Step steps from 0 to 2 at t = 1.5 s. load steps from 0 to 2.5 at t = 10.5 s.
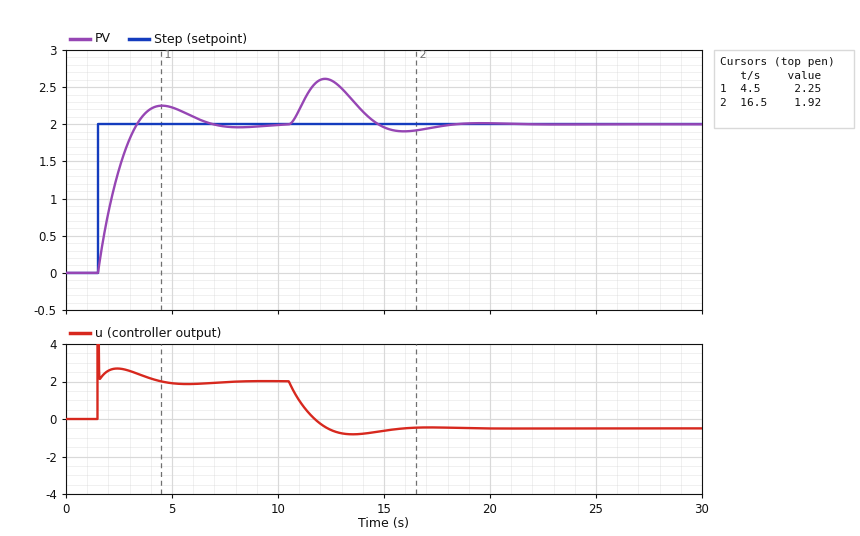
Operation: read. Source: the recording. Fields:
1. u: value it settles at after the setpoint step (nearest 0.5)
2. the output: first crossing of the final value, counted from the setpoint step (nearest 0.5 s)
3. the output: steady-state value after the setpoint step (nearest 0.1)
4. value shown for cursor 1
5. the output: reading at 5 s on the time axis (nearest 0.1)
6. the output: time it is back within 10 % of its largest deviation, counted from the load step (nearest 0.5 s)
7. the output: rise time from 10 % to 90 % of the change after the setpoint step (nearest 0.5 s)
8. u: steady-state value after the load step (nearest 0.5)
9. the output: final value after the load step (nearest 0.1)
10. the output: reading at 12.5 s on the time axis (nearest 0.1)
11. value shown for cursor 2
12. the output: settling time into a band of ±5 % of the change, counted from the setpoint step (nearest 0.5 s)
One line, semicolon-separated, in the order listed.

2.0; 2.0 s; 2.0; 2.25; 2.2; 6.5 s; 1.5 s; -0.5; 2.0; 2.6; 1.92; 4.5 s
